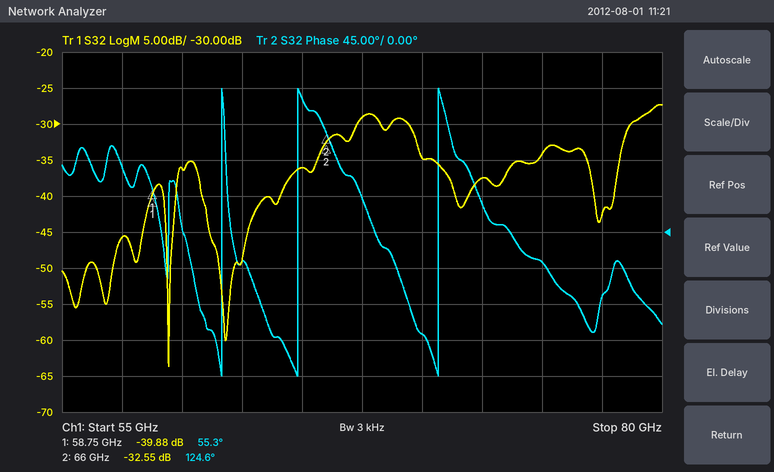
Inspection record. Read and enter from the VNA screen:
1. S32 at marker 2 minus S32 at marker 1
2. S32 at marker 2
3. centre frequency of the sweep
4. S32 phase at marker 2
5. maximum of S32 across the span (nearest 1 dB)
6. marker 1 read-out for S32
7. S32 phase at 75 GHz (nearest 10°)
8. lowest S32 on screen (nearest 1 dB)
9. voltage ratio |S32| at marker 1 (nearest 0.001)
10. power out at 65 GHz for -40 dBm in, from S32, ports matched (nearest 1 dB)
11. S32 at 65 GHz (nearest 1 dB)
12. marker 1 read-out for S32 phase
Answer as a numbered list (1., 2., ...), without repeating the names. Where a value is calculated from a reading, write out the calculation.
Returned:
1. -32.55 − (-39.88) = 7.33 dB
2. -32.55 dB
3. 67.5 GHz
4. 124.6°
5. -27 dB
6. -39.88 dB
7. -40°
8. -64 dB
9. 10^(-39.88/20) ≈ 0.010
10. -40 dBm + (-36 dB) = -76 dBm
11. -36 dB
12. 55.3°
